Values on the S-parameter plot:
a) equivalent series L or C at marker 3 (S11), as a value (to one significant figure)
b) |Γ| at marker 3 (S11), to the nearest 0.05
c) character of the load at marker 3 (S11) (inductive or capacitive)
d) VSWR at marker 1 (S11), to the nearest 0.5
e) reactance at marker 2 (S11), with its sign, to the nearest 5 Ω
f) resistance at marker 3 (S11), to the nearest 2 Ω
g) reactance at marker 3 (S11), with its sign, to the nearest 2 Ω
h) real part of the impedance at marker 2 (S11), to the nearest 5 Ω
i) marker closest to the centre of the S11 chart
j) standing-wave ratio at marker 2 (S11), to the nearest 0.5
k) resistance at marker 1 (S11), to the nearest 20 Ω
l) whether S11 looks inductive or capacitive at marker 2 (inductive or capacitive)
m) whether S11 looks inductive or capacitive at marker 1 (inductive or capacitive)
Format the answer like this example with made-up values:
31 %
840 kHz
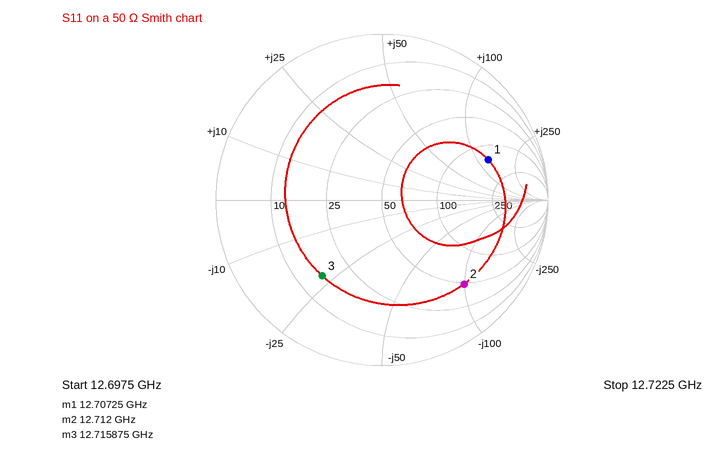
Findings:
600 fF
0.60
capacitive
5.5
-100 Ω
16 Ω
-22 Ω
50 Ω
marker 3
6.0
140 Ω
capacitive
inductive
